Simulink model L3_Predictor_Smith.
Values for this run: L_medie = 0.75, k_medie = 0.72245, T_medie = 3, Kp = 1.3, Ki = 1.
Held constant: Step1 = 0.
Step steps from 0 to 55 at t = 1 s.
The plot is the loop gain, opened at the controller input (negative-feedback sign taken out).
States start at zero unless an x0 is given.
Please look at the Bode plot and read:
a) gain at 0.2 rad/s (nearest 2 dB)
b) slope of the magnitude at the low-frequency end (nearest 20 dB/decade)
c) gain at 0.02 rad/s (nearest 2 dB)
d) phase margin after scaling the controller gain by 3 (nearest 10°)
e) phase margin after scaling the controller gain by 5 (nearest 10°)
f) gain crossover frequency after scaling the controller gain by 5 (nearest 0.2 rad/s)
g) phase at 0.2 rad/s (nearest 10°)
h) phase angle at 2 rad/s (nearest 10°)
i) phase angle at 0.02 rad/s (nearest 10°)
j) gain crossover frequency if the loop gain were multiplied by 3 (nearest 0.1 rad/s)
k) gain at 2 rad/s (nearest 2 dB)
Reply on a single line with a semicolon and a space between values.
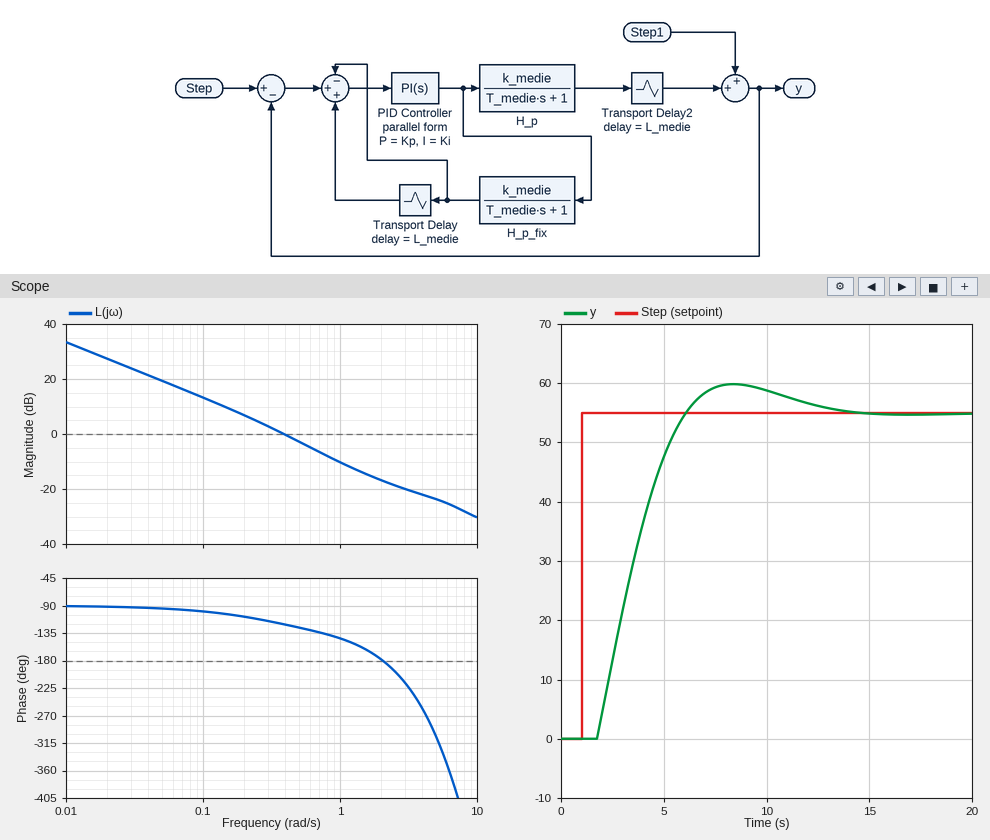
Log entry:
6 dB; -20 dB/decade; 28 dB; 40°; 20°; 1.4 rad/s; -110°; -180°; -90°; 0.9 rad/s; -16 dB
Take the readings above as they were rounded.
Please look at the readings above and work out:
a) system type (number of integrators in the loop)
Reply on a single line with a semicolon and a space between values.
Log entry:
1
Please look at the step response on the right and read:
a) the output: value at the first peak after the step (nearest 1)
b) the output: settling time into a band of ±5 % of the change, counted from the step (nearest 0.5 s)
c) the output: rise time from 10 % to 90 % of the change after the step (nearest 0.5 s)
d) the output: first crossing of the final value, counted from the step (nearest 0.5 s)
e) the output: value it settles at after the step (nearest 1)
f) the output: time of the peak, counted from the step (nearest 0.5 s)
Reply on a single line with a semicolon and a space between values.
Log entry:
60; 10.0 s; 3.0 s; 5.0 s; 55; 7.5 s
